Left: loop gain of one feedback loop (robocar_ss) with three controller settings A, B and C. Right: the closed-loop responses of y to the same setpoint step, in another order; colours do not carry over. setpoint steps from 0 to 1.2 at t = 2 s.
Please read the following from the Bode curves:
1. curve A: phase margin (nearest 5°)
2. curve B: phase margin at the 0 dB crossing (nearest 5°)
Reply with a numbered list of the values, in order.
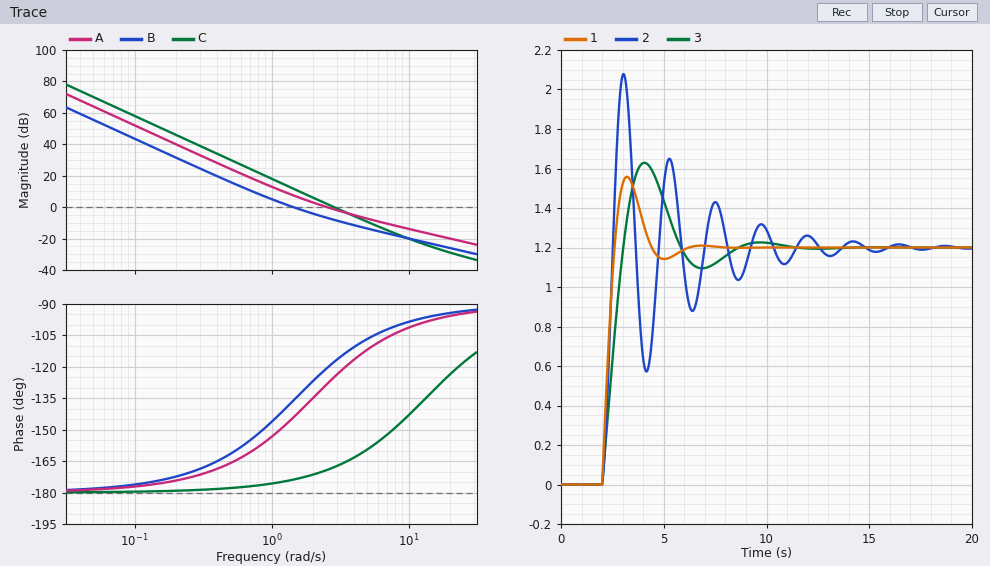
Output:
1. 50°
2. 45°
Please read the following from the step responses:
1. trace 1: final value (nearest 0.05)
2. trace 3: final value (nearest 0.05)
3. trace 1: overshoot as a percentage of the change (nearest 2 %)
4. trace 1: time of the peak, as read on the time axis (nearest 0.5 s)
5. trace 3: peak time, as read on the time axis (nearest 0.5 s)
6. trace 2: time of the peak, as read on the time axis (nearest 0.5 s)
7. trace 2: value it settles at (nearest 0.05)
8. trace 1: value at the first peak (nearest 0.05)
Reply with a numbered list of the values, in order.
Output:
1. 1.20
2. 1.20
3. 30 %
4. 3.0 s
5. 4.0 s
6. 3.0 s
7. 1.20
8. 1.55
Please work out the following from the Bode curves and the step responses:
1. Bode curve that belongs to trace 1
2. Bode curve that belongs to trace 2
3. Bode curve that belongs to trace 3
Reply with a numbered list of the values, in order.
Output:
1. A
2. C
3. B
